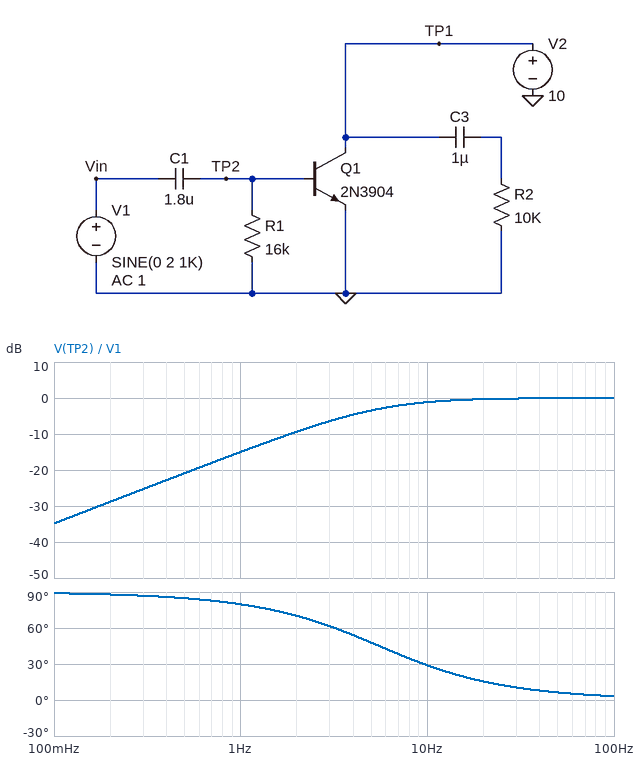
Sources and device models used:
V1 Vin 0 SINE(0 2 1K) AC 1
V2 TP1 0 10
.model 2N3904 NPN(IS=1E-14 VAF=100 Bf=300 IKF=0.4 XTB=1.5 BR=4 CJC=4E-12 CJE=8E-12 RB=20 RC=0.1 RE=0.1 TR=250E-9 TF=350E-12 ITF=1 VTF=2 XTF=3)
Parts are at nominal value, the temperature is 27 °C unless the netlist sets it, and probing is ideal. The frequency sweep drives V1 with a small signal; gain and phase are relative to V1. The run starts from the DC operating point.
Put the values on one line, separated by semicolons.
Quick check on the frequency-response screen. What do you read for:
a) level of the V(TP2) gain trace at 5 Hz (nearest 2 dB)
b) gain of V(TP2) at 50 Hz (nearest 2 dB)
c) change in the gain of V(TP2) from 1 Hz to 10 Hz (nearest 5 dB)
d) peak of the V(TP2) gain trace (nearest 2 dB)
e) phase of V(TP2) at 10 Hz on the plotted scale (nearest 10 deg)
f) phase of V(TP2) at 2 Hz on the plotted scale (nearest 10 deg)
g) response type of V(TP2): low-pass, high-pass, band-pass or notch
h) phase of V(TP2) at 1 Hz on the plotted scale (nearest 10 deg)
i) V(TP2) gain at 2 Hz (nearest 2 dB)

-4 dB; 0 dB; 15 dB; 0 dB; 30 deg; 70 deg; high-pass; 80 deg; -10 dB
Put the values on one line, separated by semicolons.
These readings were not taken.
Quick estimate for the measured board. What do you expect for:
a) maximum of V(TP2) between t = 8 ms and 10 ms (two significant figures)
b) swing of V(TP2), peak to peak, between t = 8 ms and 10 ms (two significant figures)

850 mV; 4.0 V
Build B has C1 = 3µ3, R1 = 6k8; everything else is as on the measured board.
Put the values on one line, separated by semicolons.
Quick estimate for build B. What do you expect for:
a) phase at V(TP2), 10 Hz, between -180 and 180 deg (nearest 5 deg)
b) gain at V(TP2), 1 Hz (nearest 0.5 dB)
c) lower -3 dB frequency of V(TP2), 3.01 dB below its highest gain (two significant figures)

35 deg; -17.0 dB; 7.1 Hz
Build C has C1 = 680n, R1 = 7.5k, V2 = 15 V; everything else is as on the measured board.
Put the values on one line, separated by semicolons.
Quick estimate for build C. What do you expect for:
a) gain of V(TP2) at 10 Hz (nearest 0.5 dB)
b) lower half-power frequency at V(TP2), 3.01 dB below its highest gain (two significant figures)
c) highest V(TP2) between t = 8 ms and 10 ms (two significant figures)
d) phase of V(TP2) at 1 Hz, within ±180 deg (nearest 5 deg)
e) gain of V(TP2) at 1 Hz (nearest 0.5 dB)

-10.5 dB; 31 Hz; 890 mV; 90 deg; -30.0 dB
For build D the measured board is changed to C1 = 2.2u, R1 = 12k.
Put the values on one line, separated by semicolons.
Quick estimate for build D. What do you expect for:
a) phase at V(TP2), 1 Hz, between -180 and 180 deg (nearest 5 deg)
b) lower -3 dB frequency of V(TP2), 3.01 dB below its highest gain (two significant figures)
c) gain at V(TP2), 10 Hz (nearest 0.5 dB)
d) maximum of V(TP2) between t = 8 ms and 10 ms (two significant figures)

80 deg; 6.0 Hz; -1.5 dB; 870 mV
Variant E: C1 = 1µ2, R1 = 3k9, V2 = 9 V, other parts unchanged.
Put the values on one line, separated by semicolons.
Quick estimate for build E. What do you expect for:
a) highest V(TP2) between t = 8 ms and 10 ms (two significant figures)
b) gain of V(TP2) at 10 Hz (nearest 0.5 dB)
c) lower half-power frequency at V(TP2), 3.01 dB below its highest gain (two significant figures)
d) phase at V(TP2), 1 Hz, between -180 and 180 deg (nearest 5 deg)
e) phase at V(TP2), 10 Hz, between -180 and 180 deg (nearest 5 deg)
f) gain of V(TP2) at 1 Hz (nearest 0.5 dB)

940 mV; -11.0 dB; 34 Hz; 90 deg; 75 deg; -30.5 dB
